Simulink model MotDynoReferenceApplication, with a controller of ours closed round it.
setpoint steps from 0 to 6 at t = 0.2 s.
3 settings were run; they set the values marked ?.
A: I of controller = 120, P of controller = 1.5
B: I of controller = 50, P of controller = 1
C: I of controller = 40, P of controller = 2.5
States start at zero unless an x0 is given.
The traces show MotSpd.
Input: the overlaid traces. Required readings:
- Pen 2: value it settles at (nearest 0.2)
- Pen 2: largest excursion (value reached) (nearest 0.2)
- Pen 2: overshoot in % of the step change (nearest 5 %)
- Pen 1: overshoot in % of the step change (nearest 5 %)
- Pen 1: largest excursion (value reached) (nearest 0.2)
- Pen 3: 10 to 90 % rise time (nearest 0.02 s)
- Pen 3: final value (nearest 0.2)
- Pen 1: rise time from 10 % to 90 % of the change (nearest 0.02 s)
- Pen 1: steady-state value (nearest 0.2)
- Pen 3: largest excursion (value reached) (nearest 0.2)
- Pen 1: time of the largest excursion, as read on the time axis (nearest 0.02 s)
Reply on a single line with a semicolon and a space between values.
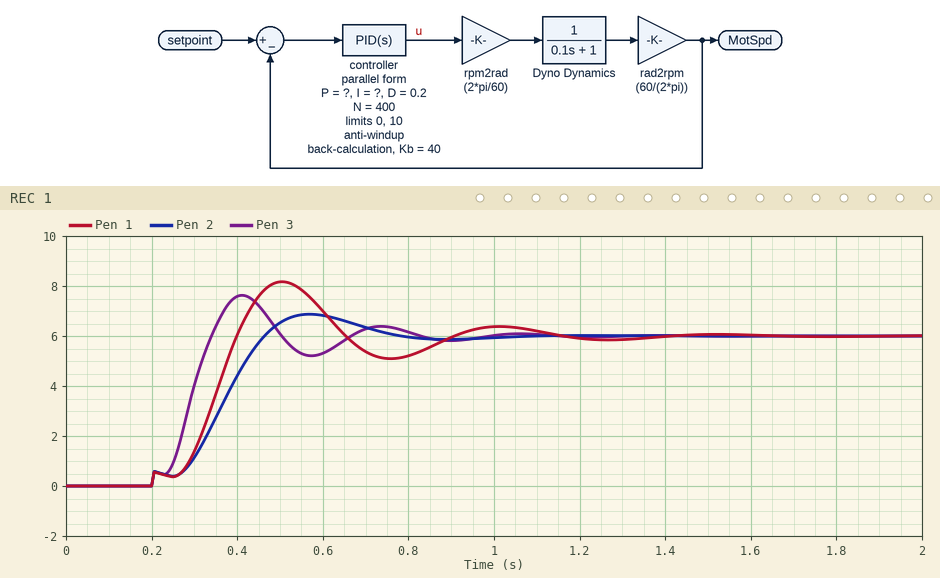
6.0; 6.8; 15 %; 35 %; 8.2; 0.08 s; 6.0; 0.12 s; 6.0; 7.6; 0.50 s
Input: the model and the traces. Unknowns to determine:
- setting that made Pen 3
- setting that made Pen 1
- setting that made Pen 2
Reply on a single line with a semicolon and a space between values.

A; B; C
